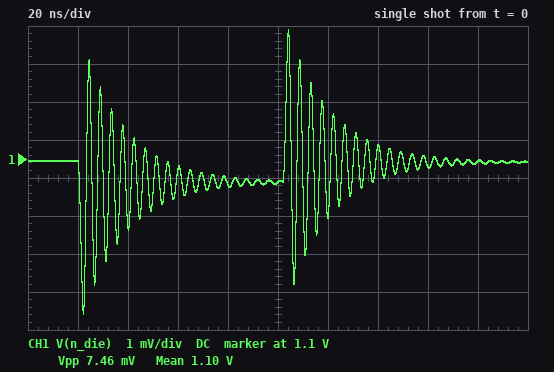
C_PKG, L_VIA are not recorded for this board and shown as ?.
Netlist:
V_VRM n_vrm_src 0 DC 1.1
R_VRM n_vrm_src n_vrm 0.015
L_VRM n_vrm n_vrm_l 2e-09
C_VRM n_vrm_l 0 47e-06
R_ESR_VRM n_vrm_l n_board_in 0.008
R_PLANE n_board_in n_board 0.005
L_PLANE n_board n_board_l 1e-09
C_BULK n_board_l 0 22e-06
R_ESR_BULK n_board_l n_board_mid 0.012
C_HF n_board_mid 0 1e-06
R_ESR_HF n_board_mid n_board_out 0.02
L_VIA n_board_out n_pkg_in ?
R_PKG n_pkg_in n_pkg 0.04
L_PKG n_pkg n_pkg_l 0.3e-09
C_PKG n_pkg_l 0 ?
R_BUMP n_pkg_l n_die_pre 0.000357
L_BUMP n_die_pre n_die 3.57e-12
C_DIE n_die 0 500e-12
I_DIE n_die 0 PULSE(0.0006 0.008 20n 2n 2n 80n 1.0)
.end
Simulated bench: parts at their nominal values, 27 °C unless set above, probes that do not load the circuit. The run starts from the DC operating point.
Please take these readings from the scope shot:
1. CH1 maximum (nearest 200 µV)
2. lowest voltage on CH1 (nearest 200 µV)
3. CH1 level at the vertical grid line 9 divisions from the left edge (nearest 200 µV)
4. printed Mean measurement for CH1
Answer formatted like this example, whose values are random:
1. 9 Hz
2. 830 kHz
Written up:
1. 1.1034 V
2. 1.0960 V
3. 1.1000 V
4. 1.10 V
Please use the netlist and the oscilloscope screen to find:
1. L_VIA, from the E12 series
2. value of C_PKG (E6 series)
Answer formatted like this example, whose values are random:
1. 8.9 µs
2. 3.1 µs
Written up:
1. 220 pH
2. 470 pF
